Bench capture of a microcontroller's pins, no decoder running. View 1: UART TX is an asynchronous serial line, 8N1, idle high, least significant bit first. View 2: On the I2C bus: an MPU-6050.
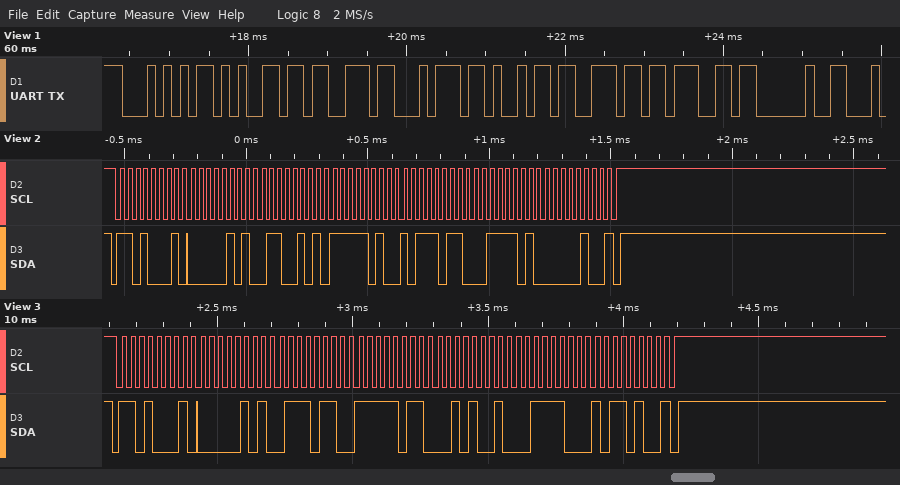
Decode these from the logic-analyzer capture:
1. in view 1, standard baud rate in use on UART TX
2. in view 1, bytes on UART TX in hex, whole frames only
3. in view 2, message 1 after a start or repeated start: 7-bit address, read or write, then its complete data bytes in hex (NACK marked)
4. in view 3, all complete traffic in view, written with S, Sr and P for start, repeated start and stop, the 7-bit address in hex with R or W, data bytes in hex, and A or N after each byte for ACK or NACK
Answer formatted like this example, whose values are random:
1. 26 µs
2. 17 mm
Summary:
1. 9600 baud
2. 54 65 73 74 69 6E 67 20
3. 0x68 read: 05 65 FA BB 3D 04 NACK
4. S 68R A 05 A 76 A FB A 29 A 3C A B4 N P
